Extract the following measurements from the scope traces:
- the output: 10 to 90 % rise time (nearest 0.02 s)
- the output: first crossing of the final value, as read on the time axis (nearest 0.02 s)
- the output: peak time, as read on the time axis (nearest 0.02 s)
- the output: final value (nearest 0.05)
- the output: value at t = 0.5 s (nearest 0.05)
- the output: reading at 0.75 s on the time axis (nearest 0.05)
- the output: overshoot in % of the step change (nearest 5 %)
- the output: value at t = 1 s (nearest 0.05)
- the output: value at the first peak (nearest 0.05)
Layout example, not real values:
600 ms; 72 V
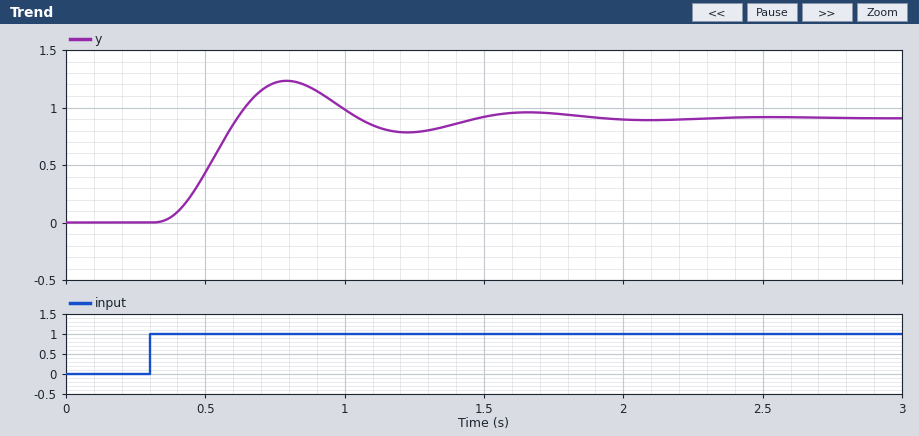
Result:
0.20 s; 0.62 s; 0.80 s; 0.90; 0.45; 1.20; 35 %; 1.00; 1.25
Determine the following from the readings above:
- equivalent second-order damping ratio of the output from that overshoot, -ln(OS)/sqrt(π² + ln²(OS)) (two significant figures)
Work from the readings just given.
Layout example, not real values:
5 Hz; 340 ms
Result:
0.32
